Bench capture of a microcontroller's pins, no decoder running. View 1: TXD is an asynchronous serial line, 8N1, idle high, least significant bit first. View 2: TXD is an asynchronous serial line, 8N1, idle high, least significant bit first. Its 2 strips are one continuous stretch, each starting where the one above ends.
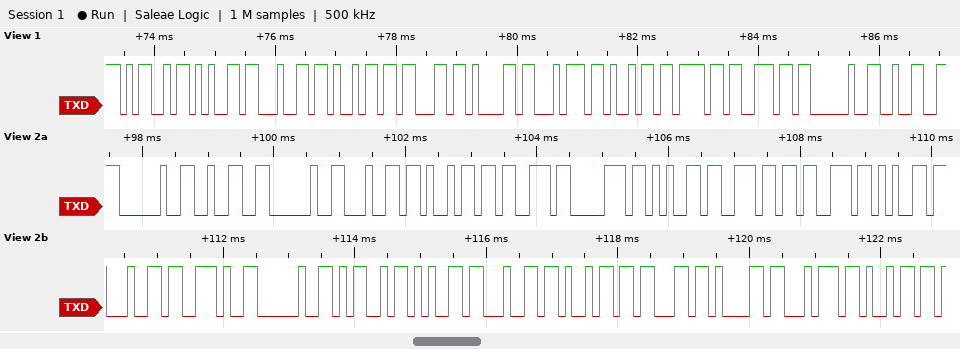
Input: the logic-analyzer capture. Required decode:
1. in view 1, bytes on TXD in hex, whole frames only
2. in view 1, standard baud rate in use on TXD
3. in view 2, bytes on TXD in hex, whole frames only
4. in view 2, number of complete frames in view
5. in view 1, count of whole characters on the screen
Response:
4D 65 64 69 63 61 74 69 6F 6E 20 32
9600 baud
20 32 20 64 69 73 70 65 6E 73 65 64 2E 20 4D 65 64 69 63 61 74 69
22
12
